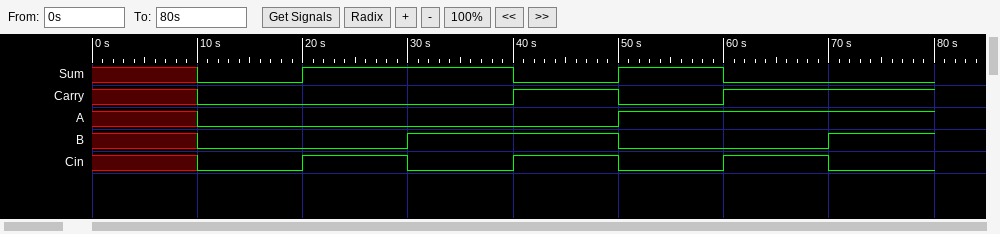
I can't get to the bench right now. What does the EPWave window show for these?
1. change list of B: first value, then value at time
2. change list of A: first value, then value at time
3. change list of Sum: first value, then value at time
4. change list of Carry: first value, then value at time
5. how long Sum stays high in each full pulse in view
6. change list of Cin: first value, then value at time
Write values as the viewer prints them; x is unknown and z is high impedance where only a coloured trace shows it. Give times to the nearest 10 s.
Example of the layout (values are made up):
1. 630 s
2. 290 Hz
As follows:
1. x, 0 at 10 s, 1 at 30 s, 0 at 50 s, 1 at 70 s
2. x, 0 at 10 s, 1 at 50 s
3. x, 0 at 10 s, 1 at 20 s, 0 at 40 s, 1 at 50 s, 0 at 60 s
4. x, 0 at 10 s, 1 at 40 s, 0 at 50 s, 1 at 60 s
5. 20 s, 10 s
6. x, 0 at 10 s, 1 at 20 s, 0 at 30 s, 1 at 40 s, 0 at 50 s, 1 at 60 s, 0 at 70 s
